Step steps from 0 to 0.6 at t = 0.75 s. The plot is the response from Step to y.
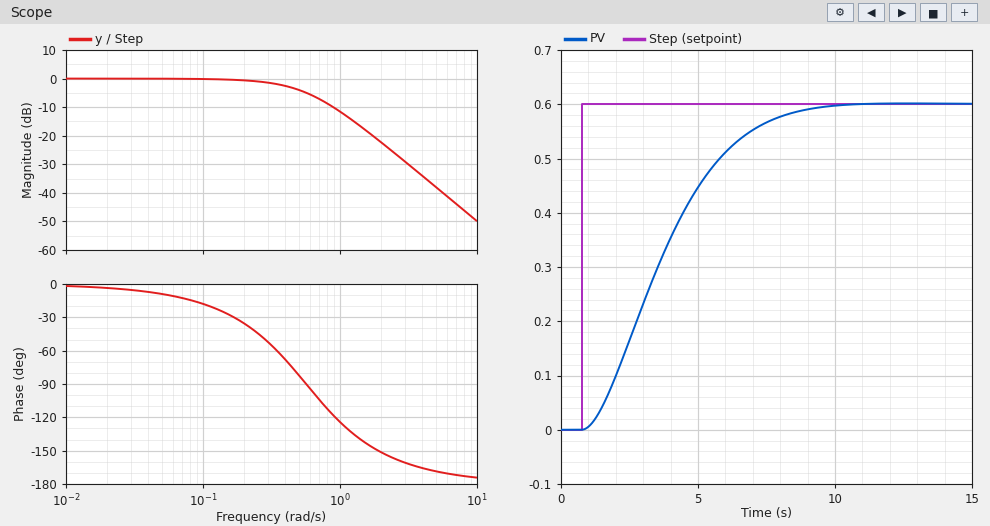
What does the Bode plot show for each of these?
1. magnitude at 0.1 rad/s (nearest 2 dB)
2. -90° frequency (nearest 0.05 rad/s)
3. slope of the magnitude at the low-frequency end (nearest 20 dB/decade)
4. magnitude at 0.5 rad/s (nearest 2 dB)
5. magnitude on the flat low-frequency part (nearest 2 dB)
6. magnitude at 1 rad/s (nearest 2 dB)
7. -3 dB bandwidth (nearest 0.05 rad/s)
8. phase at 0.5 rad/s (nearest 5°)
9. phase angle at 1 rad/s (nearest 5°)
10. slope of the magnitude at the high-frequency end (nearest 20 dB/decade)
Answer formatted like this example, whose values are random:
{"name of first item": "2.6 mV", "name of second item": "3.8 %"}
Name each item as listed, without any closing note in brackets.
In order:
{"magnitude at 0.1 rad/s": "0 dB", "-90° frequency": "0.55 rad/s", "slope of the magnitude at the low-frequency end": "0 dB/decade", "magnitude at 0.5 rad/s": "-4 dB", "magnitude on the flat low-frequency part": "0 dB", "magnitude at 1 rad/s": "-12 dB", "-3 dB bandwidth": "0.45 rad/s", "phase at 0.5 rad/s": "-80°", "phase angle at 1 rad/s": "-125°", "slope of the magnitude at the high-frequency end": "-40 dB/decade"}
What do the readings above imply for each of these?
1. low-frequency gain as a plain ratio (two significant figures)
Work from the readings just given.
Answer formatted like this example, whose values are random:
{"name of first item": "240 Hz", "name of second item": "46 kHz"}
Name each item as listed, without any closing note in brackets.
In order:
{"low-frequency gain as a plain ratio": "1.0"}
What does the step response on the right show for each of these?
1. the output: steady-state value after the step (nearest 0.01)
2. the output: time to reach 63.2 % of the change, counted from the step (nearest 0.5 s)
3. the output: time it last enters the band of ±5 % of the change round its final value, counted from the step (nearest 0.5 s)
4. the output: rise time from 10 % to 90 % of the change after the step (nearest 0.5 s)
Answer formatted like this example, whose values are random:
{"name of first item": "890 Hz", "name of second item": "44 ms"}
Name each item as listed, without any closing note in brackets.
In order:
{"the output: steady-state value after the step": "0.60", "the output: time to reach 63.2 % of the change, counted from the step": "3.5 s", "the output: time it last enters the band of ±5 % of the change round its final value, counted from the step": "7.0 s", "the output: rise time from 10 % to 90 % of the change after the step": "5.0 s"}
